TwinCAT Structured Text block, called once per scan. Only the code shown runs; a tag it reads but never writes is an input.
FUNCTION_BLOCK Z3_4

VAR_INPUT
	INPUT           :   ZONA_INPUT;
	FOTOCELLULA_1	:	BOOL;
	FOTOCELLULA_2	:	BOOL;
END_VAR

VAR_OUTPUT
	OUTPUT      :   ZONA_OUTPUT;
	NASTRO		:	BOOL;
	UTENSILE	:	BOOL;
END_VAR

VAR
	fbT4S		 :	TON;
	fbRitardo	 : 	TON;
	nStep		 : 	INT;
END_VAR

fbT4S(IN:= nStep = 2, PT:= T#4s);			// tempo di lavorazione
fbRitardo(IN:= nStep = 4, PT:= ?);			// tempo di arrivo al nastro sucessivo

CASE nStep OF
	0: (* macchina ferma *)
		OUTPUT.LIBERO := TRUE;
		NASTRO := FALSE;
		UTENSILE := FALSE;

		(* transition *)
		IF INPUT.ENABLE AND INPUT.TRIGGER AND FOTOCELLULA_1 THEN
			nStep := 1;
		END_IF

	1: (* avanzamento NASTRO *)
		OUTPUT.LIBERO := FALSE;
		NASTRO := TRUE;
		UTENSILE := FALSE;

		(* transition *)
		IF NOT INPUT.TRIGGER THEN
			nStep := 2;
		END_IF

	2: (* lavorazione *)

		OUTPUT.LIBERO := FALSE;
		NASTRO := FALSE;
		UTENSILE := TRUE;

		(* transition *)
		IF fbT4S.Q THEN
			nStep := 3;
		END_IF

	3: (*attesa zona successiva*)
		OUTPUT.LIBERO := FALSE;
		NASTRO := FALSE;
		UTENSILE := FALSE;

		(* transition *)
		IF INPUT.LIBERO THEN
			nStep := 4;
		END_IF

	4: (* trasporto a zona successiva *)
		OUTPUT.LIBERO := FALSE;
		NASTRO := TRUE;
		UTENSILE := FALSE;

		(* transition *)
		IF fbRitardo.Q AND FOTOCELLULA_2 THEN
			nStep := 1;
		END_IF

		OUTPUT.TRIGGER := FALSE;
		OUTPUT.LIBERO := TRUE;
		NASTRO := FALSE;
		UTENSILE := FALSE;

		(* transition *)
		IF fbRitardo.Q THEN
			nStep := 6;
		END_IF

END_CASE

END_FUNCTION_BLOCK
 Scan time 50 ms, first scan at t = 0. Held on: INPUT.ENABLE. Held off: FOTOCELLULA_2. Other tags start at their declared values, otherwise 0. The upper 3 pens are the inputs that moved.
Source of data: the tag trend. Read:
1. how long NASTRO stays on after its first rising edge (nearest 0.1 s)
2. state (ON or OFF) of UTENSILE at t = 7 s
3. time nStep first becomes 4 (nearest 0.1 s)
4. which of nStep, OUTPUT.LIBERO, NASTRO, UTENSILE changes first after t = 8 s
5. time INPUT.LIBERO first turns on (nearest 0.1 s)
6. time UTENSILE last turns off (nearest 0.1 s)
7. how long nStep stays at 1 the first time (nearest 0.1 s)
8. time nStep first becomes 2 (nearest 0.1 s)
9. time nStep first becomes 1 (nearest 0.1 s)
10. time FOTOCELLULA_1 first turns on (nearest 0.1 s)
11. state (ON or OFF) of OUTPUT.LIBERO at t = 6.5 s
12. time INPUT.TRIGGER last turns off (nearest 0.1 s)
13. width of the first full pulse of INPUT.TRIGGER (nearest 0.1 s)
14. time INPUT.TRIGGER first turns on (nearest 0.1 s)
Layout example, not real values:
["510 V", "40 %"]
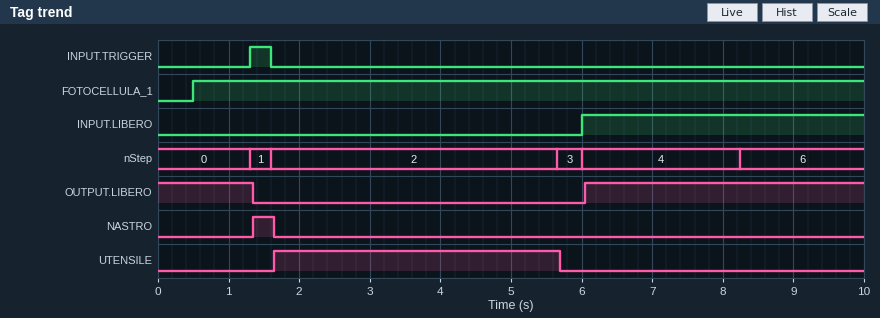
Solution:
["0.3 s", "OFF", "6.0 s", "nStep", "6.0 s", "5.7 s", "0.3 s", "1.6 s", "1.3 s", "0.5 s", "ON", "1.6 s", "0.3 s", "1.3 s"]
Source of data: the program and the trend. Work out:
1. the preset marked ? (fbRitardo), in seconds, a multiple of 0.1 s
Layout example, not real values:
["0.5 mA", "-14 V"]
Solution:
["2.2 s"]
